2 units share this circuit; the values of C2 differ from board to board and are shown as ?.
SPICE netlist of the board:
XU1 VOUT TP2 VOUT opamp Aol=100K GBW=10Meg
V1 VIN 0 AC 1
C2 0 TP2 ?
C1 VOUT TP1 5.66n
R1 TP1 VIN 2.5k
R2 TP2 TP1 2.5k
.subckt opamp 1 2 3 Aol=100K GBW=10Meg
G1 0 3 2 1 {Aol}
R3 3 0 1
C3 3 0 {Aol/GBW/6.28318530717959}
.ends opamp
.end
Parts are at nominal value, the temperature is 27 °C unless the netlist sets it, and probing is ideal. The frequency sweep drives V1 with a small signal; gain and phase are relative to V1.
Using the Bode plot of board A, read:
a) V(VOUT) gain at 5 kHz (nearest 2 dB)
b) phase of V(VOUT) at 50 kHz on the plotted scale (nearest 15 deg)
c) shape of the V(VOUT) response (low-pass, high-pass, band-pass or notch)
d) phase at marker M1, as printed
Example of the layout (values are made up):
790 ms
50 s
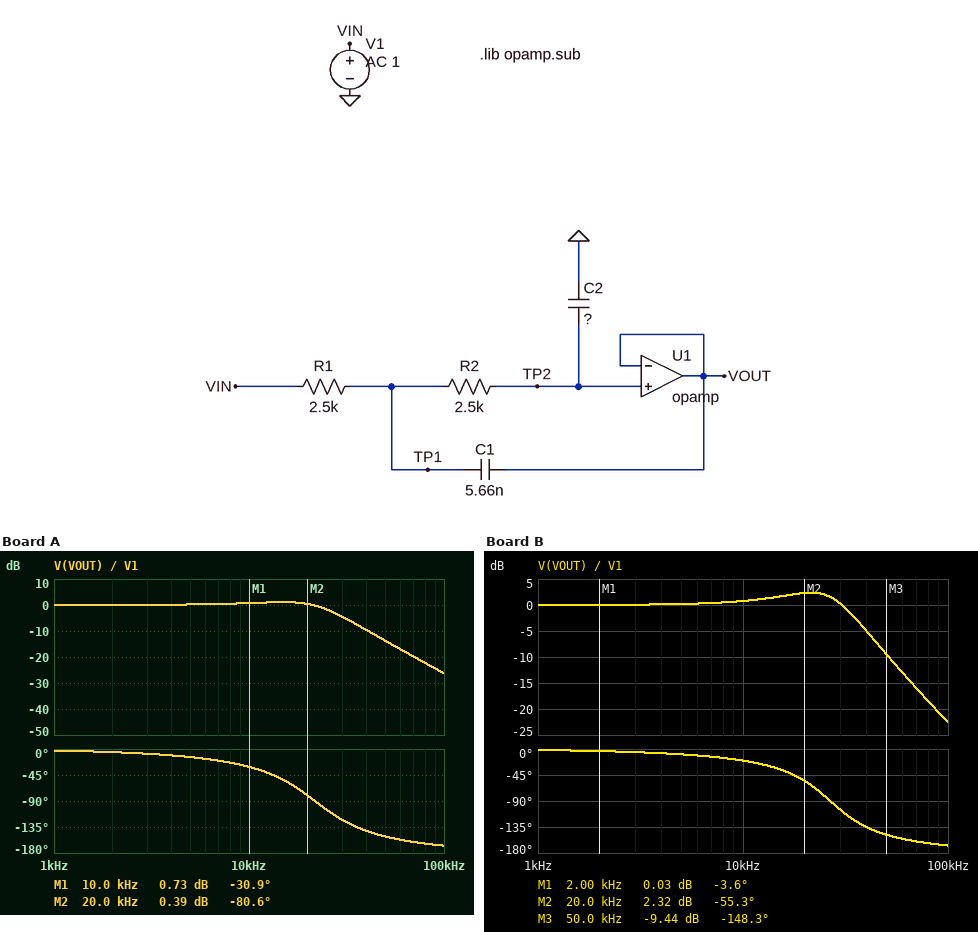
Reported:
0 dB
-150 deg
low-pass
-30.9 deg
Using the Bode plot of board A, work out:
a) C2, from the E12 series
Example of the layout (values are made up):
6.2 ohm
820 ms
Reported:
1.5 nF
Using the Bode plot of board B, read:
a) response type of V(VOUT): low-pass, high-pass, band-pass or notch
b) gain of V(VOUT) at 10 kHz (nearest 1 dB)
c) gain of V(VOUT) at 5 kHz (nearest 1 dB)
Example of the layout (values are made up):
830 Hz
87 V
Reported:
low-pass
1 dB
0 dB
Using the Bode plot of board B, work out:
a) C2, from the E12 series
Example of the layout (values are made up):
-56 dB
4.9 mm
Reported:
1 nF
